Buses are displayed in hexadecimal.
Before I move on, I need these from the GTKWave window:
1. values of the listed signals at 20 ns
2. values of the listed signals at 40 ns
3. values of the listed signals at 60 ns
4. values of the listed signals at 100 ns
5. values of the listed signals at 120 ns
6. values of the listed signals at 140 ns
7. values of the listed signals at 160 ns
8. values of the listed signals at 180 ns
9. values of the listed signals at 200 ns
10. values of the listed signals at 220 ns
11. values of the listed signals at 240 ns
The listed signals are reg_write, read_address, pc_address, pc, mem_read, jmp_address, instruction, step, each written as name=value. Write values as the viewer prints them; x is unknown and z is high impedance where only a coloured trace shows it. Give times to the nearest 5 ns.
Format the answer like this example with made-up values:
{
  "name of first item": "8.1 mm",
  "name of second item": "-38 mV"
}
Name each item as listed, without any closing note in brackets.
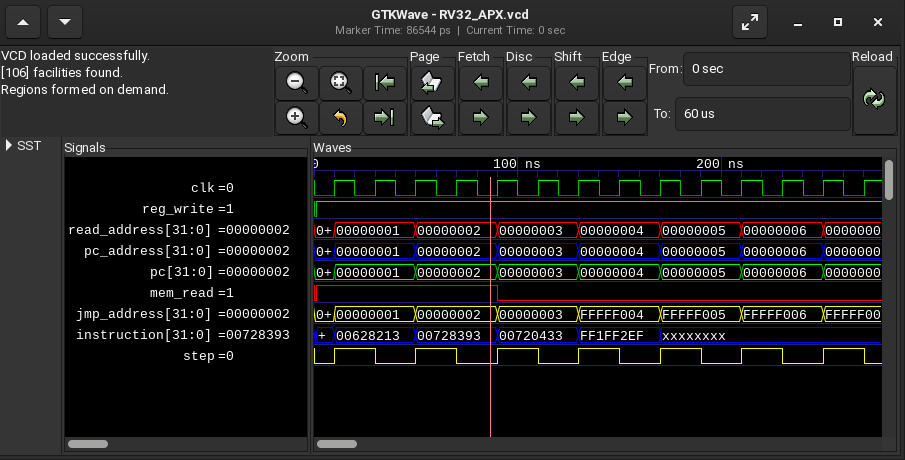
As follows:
{
  "values of the listed signals at 20 ns": "reg_write=1, read_address=00000001, pc_address=00000001, pc=00000001, mem_read=1, jmp_address=00000001, instruction=00628213, step=1",
  "values of the listed signals at 40 ns": "reg_write=1, read_address=00000001, pc_address=00000001, pc=00000001, mem_read=1, jmp_address=00000001, instruction=00628213, step=0",
  "values of the listed signals at 60 ns": "reg_write=1, read_address=00000002, pc_address=00000002, pc=00000002, mem_read=1, jmp_address=00000002, instruction=00728393, step=1",
  "values of the listed signals at 100 ns": "reg_write=1, read_address=00000003, pc_address=00000003, pc=00000003, mem_read=0, jmp_address=00000003, instruction=00720433, step=1",
  "values of the listed signals at 120 ns": "reg_write=1, read_address=00000003, pc_address=00000003, pc=00000003, mem_read=0, jmp_address=00000003, instruction=00720433, step=0",
  "values of the listed signals at 140 ns": "reg_write=1, read_address=00000004, pc_address=00000004, pc=00000004, mem_read=0, jmp_address=FFFFF004, instruction=FF1FF2EF, step=1",
  "values of the listed signals at 160 ns": "reg_write=1, read_address=00000004, pc_address=00000004, pc=00000004, mem_read=0, jmp_address=FFFFF004, instruction=FF1FF2EF, step=0",
  "values of the listed signals at 180 ns": "reg_write=1, read_address=00000005, pc_address=00000005, pc=00000005, mem_read=0, jmp_address=FFFFF005, instruction=xxxxxxxx, step=1",
  "values of the listed signals at 200 ns": "reg_write=1, read_address=00000005, pc_address=00000005, pc=00000005, mem_read=0, jmp_address=FFFFF005, instruction=xxxxxxxx, step=0",
  "values of the listed signals at 220 ns": "reg_write=1, read_address=00000006, pc_address=00000006, pc=00000006, mem_read=0, jmp_address=FFFFF006, instruction=xxxxxxxx, step=1",
  "values of the listed signals at 240 ns": "reg_write=1, read_address=00000006, pc_address=00000006, pc=00000006, mem_read=0, jmp_address=FFFFF006, instruction=xxxxxxxx, step=0"
}
